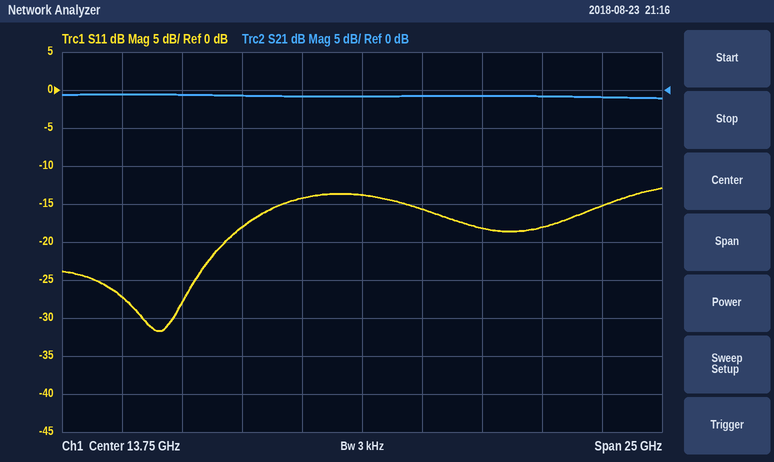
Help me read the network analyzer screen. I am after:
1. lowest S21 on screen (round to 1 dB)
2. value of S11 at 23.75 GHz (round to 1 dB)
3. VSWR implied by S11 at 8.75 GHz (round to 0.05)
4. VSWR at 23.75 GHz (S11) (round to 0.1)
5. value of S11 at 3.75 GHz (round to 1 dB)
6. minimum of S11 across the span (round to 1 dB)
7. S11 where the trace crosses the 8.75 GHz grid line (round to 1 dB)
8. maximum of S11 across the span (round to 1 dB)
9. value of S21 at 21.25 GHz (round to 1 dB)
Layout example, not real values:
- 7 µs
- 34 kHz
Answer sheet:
- -1 dB
- -15 dB
- 1.30
- 1.4
- -27 dB
- -32 dB
- -18 dB
- -13 dB
- -1 dB
